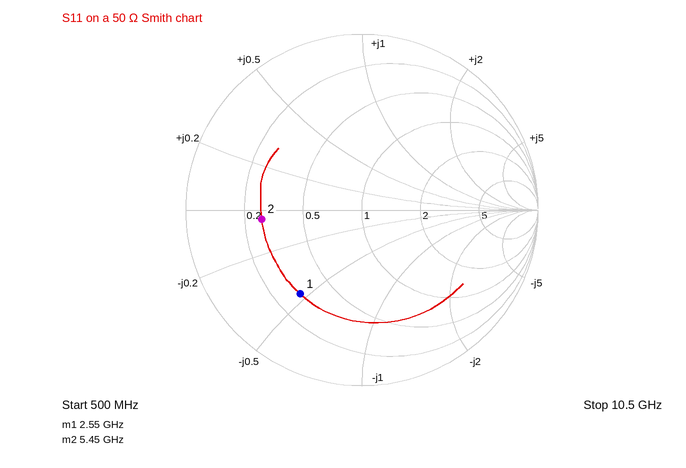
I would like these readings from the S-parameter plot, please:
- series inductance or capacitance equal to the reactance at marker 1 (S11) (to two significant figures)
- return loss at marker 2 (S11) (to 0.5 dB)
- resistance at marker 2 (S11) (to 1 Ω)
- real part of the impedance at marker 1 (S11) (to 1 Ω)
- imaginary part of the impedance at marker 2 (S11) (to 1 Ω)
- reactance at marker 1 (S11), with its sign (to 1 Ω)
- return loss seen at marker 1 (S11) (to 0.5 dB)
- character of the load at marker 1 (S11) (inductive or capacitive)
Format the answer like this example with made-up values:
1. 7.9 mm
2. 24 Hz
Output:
1. 2.7 pF
2. 5.0 dB
3. 14 Ω
4. 16 Ω
5. -2 Ω
6. -23 Ω
7. 4.5 dB
8. capacitive
